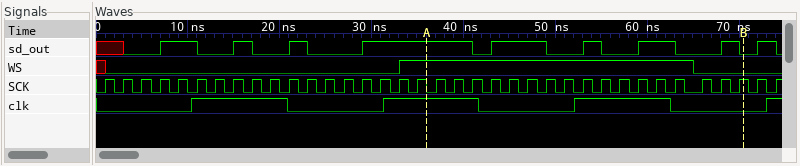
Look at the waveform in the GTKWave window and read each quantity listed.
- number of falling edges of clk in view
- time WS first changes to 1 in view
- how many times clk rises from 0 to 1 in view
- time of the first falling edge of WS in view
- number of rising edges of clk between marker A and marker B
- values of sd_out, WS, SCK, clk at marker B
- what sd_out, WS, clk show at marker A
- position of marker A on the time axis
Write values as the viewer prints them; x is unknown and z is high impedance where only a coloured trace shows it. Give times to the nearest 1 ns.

3
33 ns
4
65 ns
1
sd_out=0, WS=0, SCK=1, clk=0
sd_out=1, WS=1, clk=1
36 ns
